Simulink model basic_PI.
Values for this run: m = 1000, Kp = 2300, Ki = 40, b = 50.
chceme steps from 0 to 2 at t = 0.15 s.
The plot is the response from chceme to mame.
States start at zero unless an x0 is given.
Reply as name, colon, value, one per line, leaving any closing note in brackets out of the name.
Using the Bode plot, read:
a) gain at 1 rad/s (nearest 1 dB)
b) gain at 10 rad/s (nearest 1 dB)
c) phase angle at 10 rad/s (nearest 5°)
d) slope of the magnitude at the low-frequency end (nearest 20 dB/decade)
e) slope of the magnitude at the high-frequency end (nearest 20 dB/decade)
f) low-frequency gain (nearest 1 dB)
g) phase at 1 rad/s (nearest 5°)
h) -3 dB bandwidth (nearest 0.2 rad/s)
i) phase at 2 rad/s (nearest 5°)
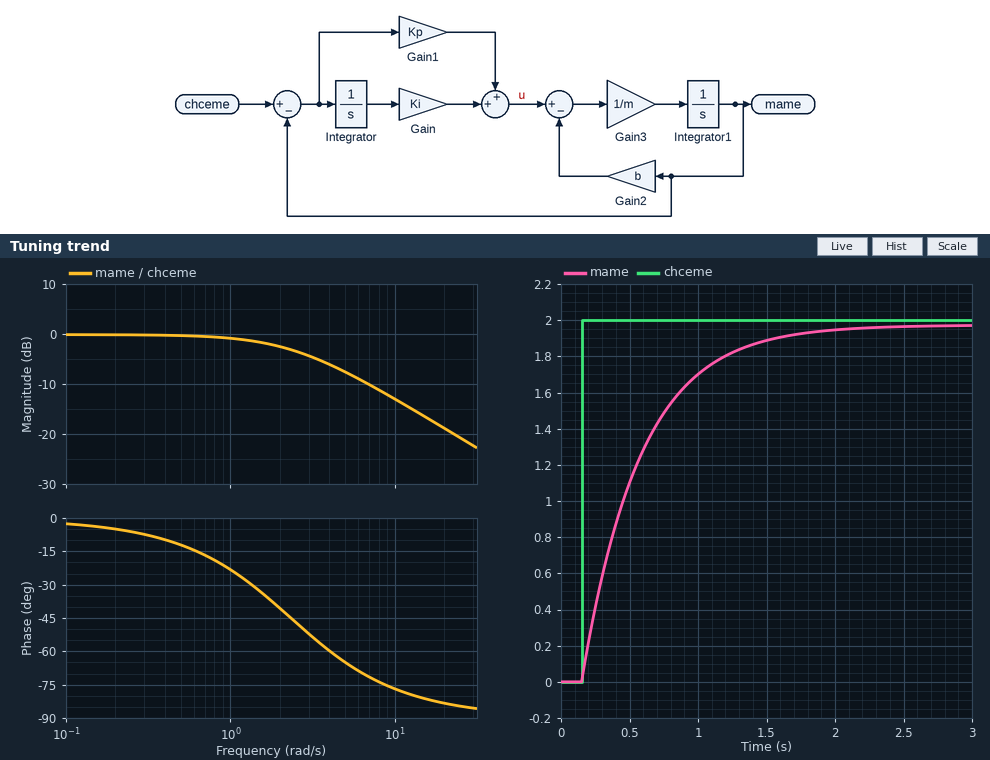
gain at 1 rad/s: -1 dB
gain at 10 rad/s: -13 dB
phase angle at 10 rad/s: -75°
slope of the magnitude at the low-frequency end: 0 dB/decade
slope of the magnitude at the high-frequency end: -20 dB/decade
low-frequency gain: 0 dB
phase at 1 rad/s: -25°
-3 dB bandwidth: 2.4 rad/s
phase at 2 rad/s: -40°
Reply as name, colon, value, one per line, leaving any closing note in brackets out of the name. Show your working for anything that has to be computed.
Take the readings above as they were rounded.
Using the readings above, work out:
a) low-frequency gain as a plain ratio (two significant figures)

low-frequency gain as a plain ratio: 10^(0 / 20) = 1.0
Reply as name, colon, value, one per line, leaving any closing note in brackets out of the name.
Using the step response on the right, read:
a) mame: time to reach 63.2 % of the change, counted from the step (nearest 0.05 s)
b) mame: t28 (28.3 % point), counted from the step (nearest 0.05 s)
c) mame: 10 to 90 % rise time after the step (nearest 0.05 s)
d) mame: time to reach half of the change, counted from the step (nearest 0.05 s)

mame: time to reach 63.2 % of the change, counted from the step: 0.45 s
mame: t28 (28.3 % point), counted from the step: 0.15 s
mame: 10 to 90 % rise time after the step: 0.95 s
mame: time to reach half of the change, counted from the step: 0.30 s
